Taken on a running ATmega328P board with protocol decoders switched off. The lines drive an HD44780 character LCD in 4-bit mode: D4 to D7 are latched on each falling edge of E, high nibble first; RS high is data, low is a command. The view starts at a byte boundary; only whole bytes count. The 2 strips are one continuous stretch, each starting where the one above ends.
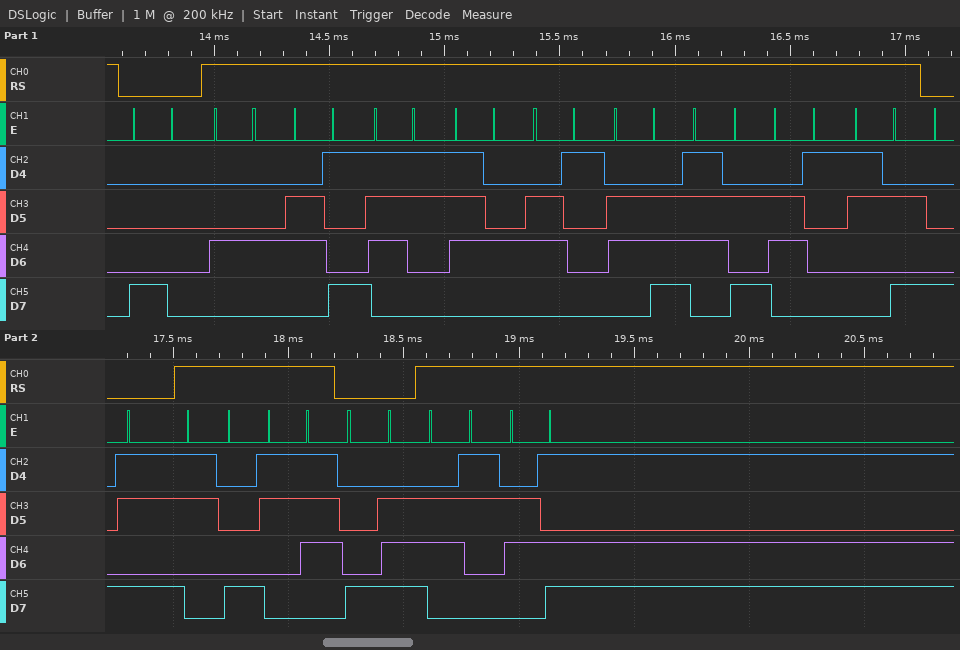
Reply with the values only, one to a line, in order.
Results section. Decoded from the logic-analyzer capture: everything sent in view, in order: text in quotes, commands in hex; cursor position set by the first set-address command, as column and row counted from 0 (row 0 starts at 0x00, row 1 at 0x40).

0x80 "Distanza:" 0x8B "87" 0x8E "cm"
column 0, row 0
